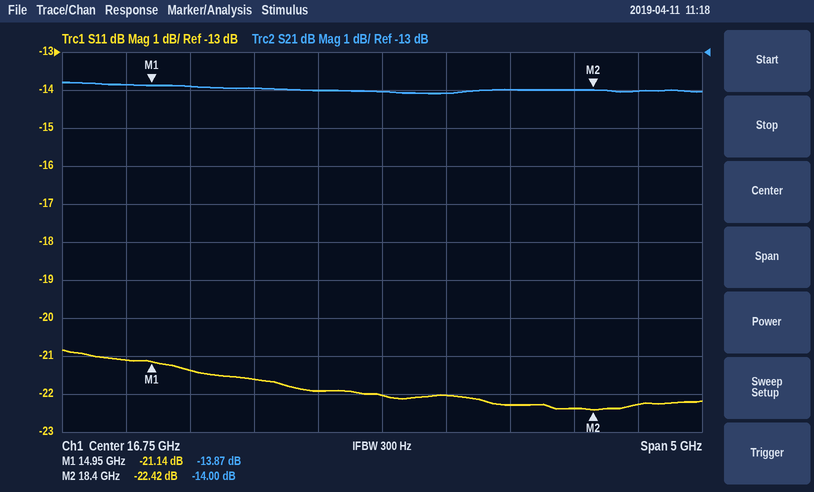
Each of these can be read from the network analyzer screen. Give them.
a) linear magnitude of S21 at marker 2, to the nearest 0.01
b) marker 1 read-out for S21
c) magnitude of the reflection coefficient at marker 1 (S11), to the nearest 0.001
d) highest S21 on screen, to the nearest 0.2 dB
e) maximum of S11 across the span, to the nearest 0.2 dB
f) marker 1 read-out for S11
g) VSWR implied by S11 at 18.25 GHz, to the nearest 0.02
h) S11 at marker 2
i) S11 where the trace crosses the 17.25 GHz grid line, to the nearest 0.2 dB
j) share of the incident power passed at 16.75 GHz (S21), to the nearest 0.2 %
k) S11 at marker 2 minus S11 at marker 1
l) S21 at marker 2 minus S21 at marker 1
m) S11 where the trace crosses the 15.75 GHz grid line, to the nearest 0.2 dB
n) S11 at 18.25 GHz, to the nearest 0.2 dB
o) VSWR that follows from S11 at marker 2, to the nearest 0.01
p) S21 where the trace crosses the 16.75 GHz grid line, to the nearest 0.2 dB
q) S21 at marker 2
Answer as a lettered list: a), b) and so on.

a) 0.20
b) -13.87 dB
c) 0.088
d) -13.8 dB
e) -20.8 dB
f) -21.14 dB
g) 1.16
h) -22.42 dB
i) -22.0 dB
j) 4.0 %
k) -1.28 dB
l) -0.13 dB
m) -21.6 dB
n) -22.4 dB
o) 1.16
p) -14.0 dB
q) -14.00 dB
